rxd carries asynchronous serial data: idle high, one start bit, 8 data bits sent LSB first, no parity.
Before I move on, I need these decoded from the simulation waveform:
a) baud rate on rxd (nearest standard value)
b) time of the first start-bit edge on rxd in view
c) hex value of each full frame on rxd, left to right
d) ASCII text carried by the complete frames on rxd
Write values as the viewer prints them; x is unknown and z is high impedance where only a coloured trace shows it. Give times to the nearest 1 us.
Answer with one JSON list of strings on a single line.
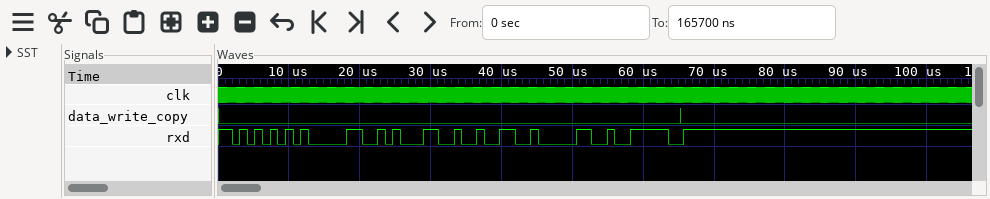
["921600 baud", "2 us", "55, 30, 31, 32, 30, 3E", "\"U0120>\""]
